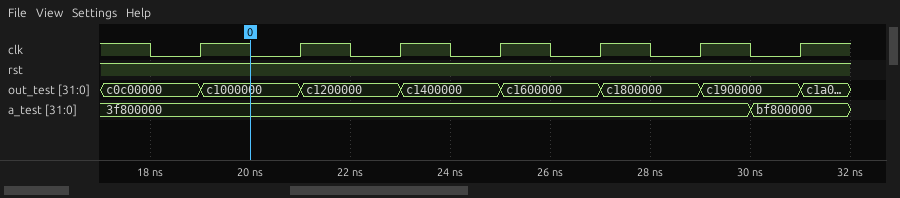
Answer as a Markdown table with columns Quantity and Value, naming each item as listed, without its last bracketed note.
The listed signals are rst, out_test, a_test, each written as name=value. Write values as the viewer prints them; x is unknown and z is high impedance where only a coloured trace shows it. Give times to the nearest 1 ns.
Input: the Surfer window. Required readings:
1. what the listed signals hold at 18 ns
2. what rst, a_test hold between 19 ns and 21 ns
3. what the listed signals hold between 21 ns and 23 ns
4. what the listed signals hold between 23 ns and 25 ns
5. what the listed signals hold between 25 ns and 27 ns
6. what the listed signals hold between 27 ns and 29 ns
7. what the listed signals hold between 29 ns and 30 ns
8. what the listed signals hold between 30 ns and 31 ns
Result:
| Quantity | Value |
|---|---|
| what the listed signals hold at 18 ns | rst=1, out_test=c0c00000, a_test=3f800000 |
| what rst, a_test hold between 19 ns and 21 ns | rst=1, a_test=3f800000 |
| what the listed signals hold between 21 ns and 23 ns | rst=1, out_test=c1200000, a_test=3f800000 |
| what the listed signals hold between 23 ns and 25 ns | rst=1, out_test=c1400000, a_test=3f800000 |
| what the listed signals hold between 25 ns and 27 ns | rst=1, out_test=c1600000, a_test=3f800000 |
| what the listed signals hold between 27 ns and 29 ns | rst=1, out_test=c1800000, a_test=3f800000 |
| what the listed signals hold between 29 ns and 30 ns | rst=1, out_test=c1900000, a_test=3f800000 |
| what the listed signals hold between 30 ns and 31 ns | rst=1, out_test=c1900000, a_test=bf800000 |
